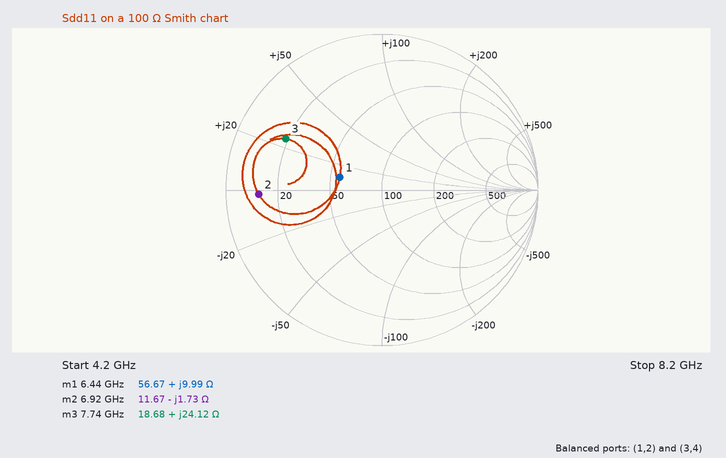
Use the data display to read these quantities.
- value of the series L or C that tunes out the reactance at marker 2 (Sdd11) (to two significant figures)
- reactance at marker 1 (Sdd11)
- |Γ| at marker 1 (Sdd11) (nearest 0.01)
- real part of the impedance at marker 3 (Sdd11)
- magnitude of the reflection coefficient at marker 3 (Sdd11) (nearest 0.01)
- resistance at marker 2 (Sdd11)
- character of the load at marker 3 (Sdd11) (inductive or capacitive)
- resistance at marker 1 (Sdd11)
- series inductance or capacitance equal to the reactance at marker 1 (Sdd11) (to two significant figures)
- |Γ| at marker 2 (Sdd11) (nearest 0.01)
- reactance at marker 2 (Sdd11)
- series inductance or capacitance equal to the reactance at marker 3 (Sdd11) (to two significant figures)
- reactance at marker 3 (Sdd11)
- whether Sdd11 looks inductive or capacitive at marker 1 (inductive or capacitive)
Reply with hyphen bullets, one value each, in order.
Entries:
- 40 pH
- +9.99 Ω
- 0.28
- 18.68 Ω
- 0.70
- 11.67 Ω
- inductive
- 56.67 Ω
- 250 pH
- 0.79
- -1.73 Ω
- 500 pH
- +24.12 Ω
- inductive
